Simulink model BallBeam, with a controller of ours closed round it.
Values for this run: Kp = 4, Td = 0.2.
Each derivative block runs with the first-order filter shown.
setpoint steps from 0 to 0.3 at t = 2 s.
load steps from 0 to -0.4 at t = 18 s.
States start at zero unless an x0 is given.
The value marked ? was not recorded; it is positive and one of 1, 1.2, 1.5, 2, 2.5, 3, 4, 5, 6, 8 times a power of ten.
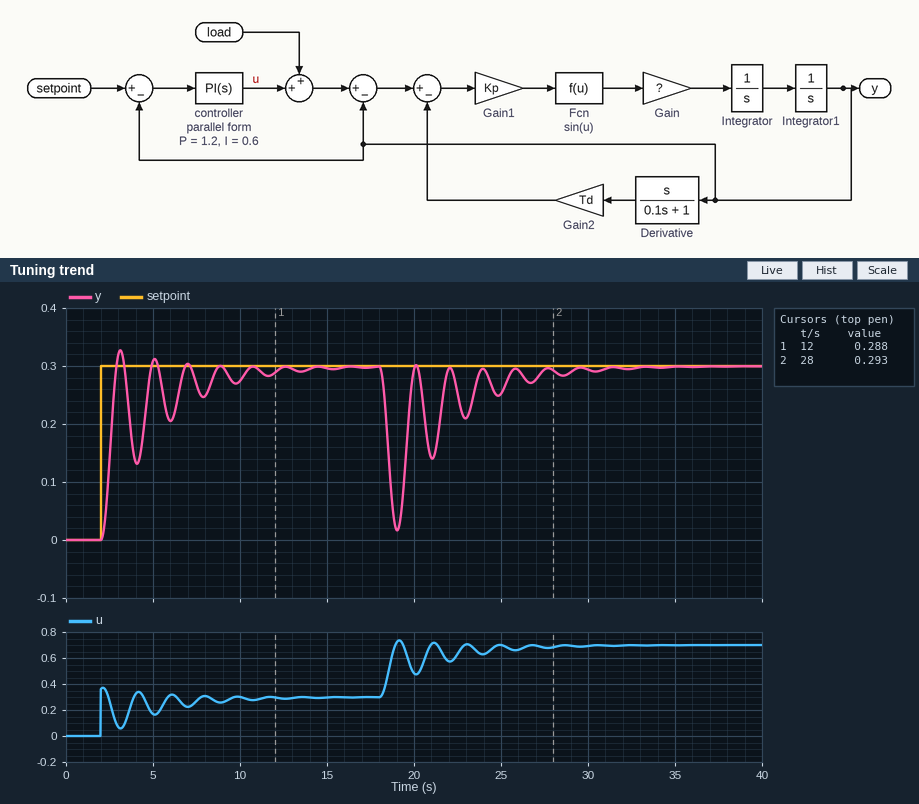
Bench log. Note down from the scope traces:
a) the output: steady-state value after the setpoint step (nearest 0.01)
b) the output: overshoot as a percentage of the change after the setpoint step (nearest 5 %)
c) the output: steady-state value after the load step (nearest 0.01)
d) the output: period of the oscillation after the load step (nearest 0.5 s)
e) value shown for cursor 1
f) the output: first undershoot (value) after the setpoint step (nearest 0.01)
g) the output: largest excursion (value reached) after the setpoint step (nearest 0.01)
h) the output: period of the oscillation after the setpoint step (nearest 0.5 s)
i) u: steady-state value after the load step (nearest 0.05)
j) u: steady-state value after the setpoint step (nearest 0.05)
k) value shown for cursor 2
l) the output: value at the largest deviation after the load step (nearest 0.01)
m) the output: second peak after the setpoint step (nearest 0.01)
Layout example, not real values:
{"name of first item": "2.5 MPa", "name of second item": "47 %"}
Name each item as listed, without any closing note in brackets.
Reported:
{"the output: steady-state value after the setpoint step": "0.30", "the output: overshoot as a percentage of the change after the setpoint step": "10 %", "the output: steady-state value after the load step": "0.30", "the output: period of the oscillation after the load step": "2.0 s", "value shown for cursor 1": "0.288", "the output: first undershoot (value) after the setpoint step": "0.13", "the output: largest excursion (value reached) after the setpoint step": "0.33", "the output: period of the oscillation after the setpoint step": "2.0 s", "u: steady-state value after the load step": "0.70", "u: steady-state value after the setpoint step": "0.30", "value shown for cursor 2": "0.293", "the output: value at the largest deviation after the load step": "0.02", "the output: second peak after the setpoint step": "0.31"}
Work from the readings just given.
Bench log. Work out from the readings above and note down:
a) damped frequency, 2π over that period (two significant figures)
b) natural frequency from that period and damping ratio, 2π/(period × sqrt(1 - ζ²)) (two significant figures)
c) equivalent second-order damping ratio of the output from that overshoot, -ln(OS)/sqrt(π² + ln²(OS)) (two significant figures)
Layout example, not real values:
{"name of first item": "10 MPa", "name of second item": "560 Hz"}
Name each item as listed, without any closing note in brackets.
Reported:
{"damped frequency, 2π over that period": "3.1 rad/s", "natural frequency from that period and damping ratio, 2π/(period × sqrt(1 - ζ²))": "3.9 rad/s", "equivalent second-order damping ratio of the output from that overshoot, -ln(OS)/sqrt(π² + ln²(OS))": "0.59"}
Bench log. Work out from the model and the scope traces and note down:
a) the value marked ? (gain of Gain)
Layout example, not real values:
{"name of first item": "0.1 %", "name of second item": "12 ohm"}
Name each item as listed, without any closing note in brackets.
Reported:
{"the value marked ?": "1.2"}
